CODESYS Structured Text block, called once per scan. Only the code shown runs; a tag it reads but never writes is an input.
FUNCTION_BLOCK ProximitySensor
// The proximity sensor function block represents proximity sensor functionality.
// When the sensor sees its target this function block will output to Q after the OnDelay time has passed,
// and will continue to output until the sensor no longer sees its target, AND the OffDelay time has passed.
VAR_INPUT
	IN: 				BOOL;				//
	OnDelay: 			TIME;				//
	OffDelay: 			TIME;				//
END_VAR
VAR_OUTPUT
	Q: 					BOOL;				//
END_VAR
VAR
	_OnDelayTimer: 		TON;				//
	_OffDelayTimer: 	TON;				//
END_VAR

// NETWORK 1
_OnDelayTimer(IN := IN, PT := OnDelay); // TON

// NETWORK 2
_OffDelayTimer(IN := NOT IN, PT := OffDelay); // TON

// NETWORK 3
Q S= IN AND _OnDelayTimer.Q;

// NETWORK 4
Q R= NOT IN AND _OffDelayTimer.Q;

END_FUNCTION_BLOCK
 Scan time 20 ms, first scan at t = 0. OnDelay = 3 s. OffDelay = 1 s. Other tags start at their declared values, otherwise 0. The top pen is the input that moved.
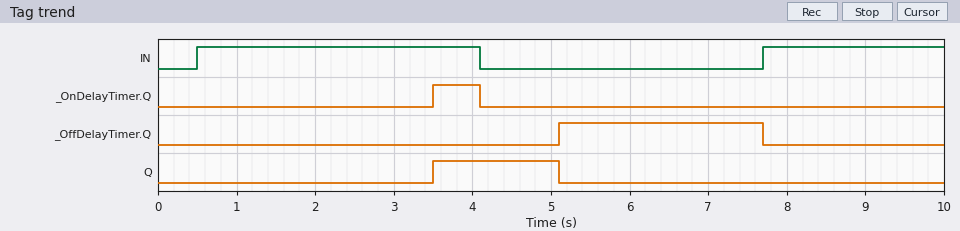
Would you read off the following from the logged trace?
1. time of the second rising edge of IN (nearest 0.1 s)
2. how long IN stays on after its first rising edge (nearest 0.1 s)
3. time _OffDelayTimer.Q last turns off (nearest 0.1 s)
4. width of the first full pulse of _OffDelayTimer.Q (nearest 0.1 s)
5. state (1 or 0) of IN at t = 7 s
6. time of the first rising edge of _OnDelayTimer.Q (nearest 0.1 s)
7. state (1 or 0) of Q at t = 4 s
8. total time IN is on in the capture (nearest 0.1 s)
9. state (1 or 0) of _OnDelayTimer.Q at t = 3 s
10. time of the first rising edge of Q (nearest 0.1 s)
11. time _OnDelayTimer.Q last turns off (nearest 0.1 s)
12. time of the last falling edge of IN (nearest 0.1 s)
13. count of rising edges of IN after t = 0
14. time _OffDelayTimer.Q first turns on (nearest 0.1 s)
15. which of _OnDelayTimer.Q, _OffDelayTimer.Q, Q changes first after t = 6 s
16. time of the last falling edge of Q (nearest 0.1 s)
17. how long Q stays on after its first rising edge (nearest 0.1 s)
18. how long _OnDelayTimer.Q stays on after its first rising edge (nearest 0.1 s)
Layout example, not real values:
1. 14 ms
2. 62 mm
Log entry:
1. 7.7 s
2. 3.6 s
3. 7.7 s
4. 2.6 s
5. 0
6. 3.5 s
7. 1
8. 5.9 s
9. 0
10. 3.5 s
11. 4.1 s
12. 4.1 s
13. 2
14. 5.1 s
15. _OffDelayTimer.Q
16. 5.1 s
17. 1.6 s
18. 0.6 s
